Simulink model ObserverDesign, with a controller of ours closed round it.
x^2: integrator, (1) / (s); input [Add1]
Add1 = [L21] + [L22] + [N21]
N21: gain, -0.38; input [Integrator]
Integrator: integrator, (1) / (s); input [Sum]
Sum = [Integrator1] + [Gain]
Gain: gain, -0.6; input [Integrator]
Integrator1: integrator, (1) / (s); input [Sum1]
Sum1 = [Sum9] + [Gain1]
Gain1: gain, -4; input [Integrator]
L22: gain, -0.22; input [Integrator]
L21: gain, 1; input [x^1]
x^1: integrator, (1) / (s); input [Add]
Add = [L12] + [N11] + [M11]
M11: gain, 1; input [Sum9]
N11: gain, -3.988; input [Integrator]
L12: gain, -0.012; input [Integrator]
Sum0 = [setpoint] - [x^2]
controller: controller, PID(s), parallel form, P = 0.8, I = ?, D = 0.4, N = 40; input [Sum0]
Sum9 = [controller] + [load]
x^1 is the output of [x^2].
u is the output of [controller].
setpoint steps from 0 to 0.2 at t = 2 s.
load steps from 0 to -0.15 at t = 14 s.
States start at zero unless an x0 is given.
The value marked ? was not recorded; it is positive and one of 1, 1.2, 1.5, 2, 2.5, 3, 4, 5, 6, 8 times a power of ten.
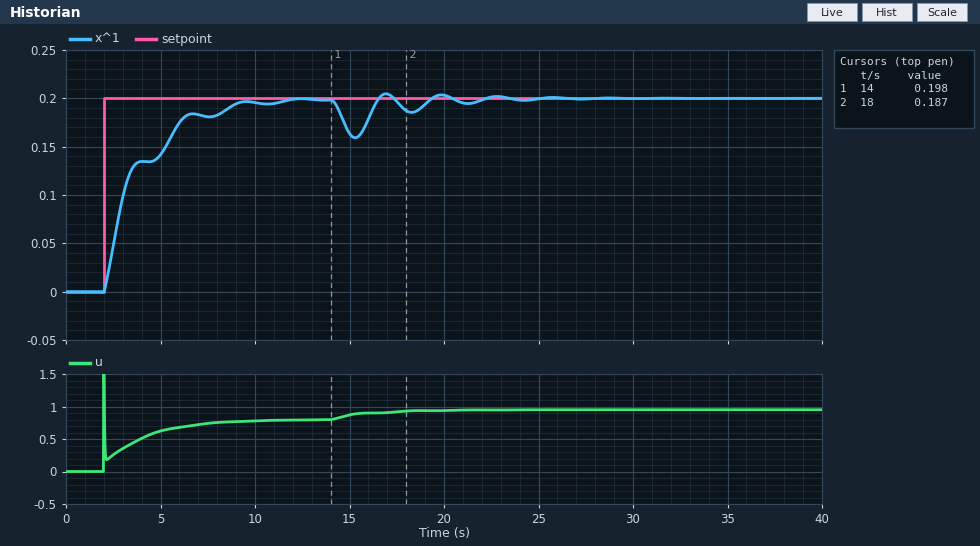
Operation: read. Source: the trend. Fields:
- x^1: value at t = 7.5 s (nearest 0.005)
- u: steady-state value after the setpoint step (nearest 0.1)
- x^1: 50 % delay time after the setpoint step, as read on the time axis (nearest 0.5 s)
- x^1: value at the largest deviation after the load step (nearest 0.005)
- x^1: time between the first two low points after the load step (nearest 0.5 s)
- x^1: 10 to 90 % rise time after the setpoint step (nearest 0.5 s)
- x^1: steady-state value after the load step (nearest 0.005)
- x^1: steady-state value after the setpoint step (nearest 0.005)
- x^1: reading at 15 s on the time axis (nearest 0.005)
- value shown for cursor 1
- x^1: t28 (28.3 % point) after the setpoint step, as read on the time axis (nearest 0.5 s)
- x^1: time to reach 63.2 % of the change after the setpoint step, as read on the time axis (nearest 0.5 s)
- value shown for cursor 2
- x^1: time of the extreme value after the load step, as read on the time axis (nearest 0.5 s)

0.180
0.8
3.0 s
0.160
3.0 s
4.0 s
0.200
0.200
0.165
0.198
2.5 s
3.5 s
0.187
15.5 s
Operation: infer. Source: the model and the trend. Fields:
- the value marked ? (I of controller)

2
